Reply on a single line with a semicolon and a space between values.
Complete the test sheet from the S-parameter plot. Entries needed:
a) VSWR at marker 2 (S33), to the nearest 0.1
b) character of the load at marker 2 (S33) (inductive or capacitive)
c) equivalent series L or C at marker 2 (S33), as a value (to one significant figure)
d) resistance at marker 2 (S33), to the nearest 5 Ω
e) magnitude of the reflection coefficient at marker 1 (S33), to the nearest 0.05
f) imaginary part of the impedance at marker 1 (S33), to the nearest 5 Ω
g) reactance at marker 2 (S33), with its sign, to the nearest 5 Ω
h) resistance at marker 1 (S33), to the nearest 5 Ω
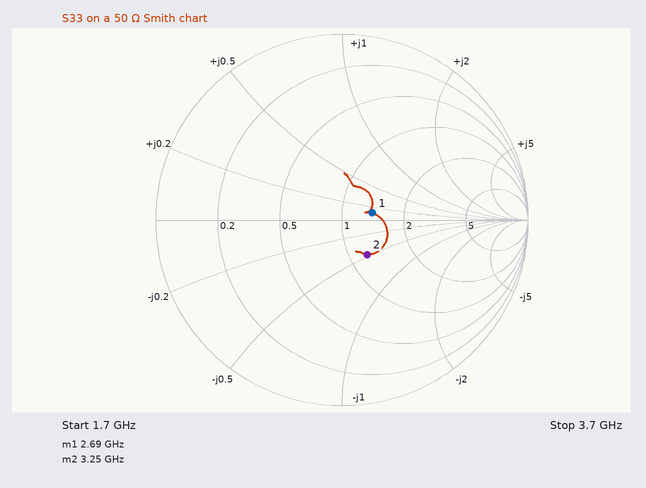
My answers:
1.6; capacitive; 2 pF; 60 Ω; 0.15; +5 Ω; -25 Ω; 70 Ω
